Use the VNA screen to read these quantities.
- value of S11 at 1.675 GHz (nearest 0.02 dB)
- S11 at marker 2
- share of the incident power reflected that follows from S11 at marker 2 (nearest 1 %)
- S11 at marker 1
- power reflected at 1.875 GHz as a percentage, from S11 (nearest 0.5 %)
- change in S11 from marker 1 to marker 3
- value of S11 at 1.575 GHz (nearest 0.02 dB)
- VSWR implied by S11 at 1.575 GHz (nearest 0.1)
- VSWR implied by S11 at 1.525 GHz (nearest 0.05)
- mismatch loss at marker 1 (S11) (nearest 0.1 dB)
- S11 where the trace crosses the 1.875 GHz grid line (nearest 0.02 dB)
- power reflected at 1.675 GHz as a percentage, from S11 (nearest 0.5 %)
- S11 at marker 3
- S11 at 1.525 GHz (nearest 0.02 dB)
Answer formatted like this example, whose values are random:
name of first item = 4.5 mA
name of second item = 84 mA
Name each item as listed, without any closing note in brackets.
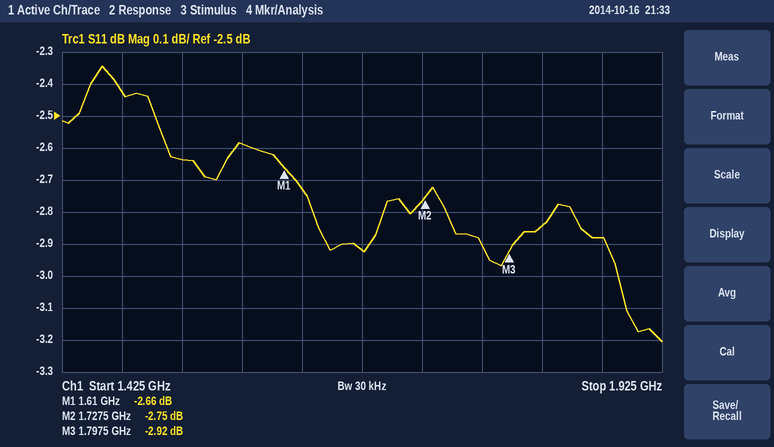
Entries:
value of S11 at 1.675 GHz = -2.92 dB
S11 at marker 2 = -2.75 dB
share of the incident power reflected that follows from S11 at marker 2 = 53 %
S11 at marker 1 = -2.66 dB
power reflected at 1.875 GHz as a percentage, from S11 = 51.5 %
change in S11 from marker 1 to marker 3 = -0.26 dB
value of S11 at 1.575 GHz = -2.58 dB
VSWR implied by S11 at 1.575 GHz = 6.8
VSWR implied by S11 at 1.525 GHz = 6.65
mismatch loss at marker 1 (S11) = 3.4 dB
S11 where the trace crosses the 1.875 GHz grid line = -2.88 dB
power reflected at 1.675 GHz as a percentage, from S11 = 51.0 %
S11 at marker 3 = -2.92 dB
S11 at 1.525 GHz = -2.64 dB
